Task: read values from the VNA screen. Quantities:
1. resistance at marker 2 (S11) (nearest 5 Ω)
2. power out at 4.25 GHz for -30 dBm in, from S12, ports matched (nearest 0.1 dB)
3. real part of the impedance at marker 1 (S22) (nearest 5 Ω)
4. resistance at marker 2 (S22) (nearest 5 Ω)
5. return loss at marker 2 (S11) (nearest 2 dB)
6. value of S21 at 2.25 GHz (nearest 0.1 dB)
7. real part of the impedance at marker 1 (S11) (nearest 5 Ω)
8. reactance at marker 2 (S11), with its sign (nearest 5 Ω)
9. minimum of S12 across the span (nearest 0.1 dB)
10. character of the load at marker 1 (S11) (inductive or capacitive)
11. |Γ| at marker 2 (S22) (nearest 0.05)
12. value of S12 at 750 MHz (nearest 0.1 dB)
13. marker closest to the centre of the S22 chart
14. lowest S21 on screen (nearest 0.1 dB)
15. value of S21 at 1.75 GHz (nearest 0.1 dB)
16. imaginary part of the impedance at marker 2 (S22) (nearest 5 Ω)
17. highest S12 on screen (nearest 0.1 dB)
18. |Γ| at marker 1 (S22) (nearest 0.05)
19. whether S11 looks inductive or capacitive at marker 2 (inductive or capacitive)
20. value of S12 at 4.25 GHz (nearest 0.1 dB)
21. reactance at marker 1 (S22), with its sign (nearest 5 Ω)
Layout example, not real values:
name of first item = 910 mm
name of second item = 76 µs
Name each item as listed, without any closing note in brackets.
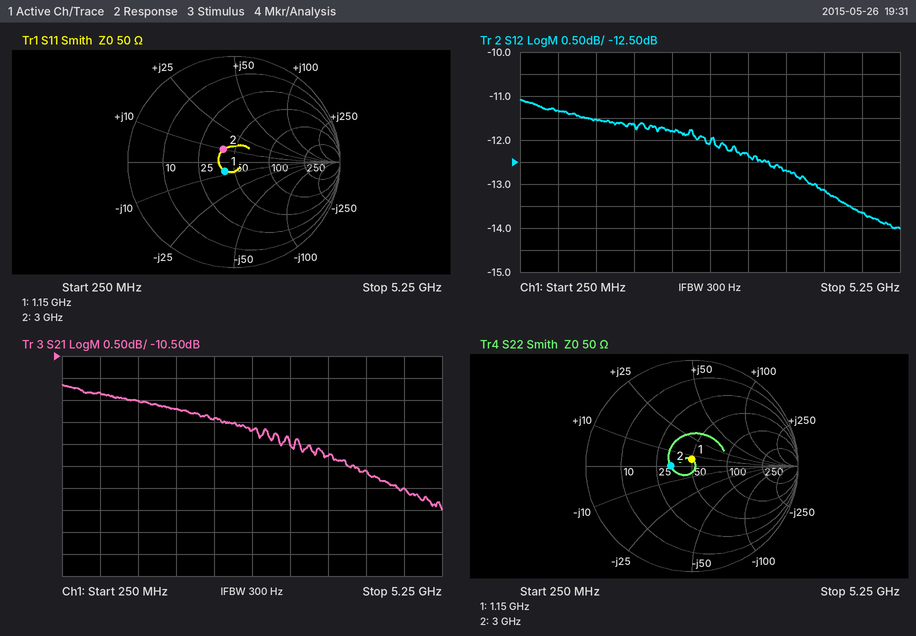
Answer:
resistance at marker 2 (S11) = 40 Ω
power out at 4.25 GHz for -30 dBm in, from S12, ports matched = -43.1 dBm
real part of the impedance at marker 1 (S22) = 50 Ω
resistance at marker 2 (S22) = 35 Ω
return loss at marker 2 (S11) = 16 dB
value of S21 at 2.25 GHz = -11.9 dB
real part of the impedance at marker 1 (S11) = 40 Ω
reactance at marker 2 (S11), with its sign = +10 Ω
minimum of S12 across the span = -14.0 dB
character of the load at marker 1 (S11) = capacitive
|Γ| at marker 2 (S22) = 0.20
value of S12 at 750 MHz = -11.3 dB
marker closest to the centre of the S22 chart = marker 1
lowest S21 on screen = -14.0 dB
value of S21 at 1.75 GHz = -11.7 dB
imaginary part of the impedance at marker 2 (S22) = 0 Ω
highest S12 on screen = -11.1 dB
|Γ| at marker 1 (S22) = 0.05
whether S11 looks inductive or capacitive at marker 2 = inductive
value of S12 at 4.25 GHz = -13.1 dB
reactance at marker 1 (S22), with its sign = +5 Ω
